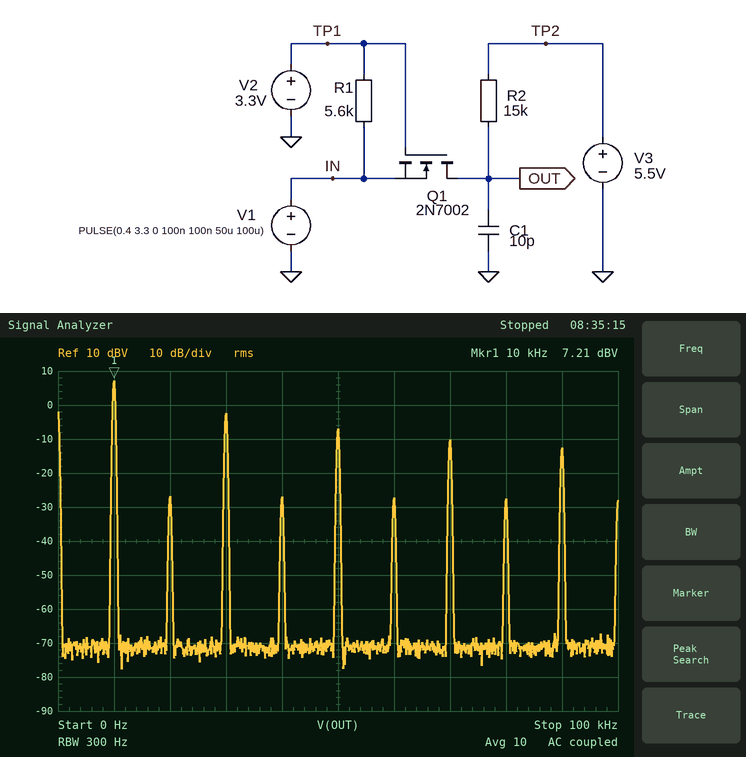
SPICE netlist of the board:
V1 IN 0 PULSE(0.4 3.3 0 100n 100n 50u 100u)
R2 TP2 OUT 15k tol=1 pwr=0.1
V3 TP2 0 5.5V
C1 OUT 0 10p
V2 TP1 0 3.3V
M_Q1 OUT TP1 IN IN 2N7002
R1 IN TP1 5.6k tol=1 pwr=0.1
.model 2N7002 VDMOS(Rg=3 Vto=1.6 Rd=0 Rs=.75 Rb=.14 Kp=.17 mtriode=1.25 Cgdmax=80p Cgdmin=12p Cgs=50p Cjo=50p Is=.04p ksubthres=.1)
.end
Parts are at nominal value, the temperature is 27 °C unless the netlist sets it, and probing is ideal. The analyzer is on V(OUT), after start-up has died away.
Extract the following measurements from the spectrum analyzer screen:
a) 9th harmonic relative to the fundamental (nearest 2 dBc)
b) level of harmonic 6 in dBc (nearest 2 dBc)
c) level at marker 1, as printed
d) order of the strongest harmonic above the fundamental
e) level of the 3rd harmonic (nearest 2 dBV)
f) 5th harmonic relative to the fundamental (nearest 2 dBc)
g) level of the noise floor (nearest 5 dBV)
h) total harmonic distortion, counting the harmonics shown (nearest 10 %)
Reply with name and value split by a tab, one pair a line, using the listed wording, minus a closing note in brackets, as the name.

9th harmonic relative to the fundamental	-20 dBc
level of harmonic 6 in dBc	-34 dBc
level at marker 1, as printed	7.21 dBV
order of the strongest harmonic above the fundamental	3
level of the 3rd harmonic	-2 dBV
5th harmonic relative to the fundamental	-14 dBc
level of the noise floor	-70 dBV
total harmonic distortion, counting the harmonics shown	40 %
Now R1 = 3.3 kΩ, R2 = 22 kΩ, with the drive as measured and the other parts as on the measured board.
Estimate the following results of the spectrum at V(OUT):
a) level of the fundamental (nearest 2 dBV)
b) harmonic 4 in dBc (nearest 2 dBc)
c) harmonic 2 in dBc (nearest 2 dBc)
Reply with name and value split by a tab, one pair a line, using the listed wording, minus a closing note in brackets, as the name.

level of the fundamental	8 dBV
harmonic 4 in dBc	-30 dBc
harmonic 2 in dBc	-30 dBc
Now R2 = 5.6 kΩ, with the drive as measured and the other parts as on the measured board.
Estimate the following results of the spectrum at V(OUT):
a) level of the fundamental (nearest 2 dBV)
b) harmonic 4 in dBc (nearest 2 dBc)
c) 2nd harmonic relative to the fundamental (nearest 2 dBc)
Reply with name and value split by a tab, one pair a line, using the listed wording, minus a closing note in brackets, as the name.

level of the fundamental	8 dBV
harmonic 4 in dBc	-44 dBc
2nd harmonic relative to the fundamental	-44 dBc
